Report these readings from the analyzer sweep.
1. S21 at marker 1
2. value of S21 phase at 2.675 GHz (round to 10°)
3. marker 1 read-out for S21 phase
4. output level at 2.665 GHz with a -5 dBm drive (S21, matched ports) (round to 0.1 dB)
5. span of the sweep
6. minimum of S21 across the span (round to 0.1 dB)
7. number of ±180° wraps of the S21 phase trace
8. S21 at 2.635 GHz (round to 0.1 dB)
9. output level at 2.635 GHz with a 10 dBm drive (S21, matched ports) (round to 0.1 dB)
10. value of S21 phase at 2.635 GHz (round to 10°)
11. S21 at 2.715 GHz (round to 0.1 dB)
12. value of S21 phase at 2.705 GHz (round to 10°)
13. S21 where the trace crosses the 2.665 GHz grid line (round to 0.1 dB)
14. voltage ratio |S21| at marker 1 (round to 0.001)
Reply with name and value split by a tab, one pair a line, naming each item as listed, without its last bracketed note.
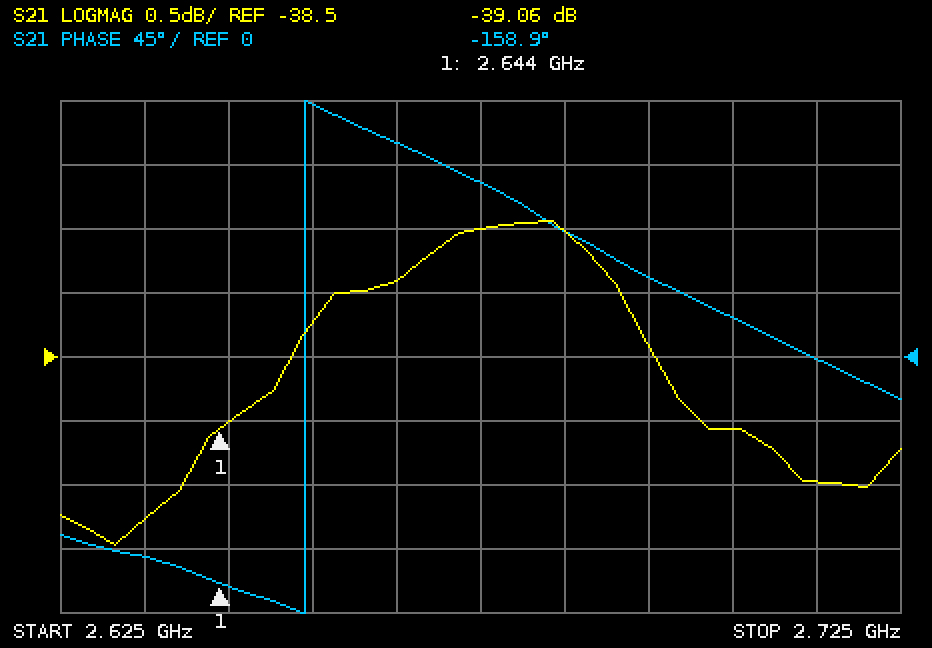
S21 at marker 1	-39.06 dB
value of S21 phase at 2.675 GHz	120°
marker 1 read-out for S21 phase	-158.9°
output level at 2.665 GHz with a -5 dBm drive (S21, matched ports)	-42.9 dBm
span of the sweep	100 MHz
minimum of S21 across the span	-40.0 dB
number of ±180° wraps of the S21 phase trace	1
S21 at 2.635 GHz	-39.8 dB
output level at 2.635 GHz with a 10 dBm drive (S21, matched ports)	-29.8 dBm
value of S21 phase at 2.635 GHz	-140°
S21 at 2.715 GHz	-39.5 dB
value of S21 phase at 2.705 GHz	30°
S21 where the trace crosses the 2.665 GHz grid line	-37.9 dB
voltage ratio |S21| at marker 1	0.011
